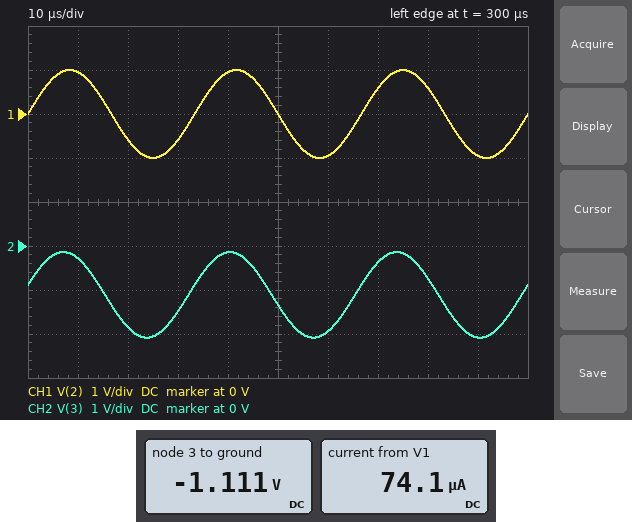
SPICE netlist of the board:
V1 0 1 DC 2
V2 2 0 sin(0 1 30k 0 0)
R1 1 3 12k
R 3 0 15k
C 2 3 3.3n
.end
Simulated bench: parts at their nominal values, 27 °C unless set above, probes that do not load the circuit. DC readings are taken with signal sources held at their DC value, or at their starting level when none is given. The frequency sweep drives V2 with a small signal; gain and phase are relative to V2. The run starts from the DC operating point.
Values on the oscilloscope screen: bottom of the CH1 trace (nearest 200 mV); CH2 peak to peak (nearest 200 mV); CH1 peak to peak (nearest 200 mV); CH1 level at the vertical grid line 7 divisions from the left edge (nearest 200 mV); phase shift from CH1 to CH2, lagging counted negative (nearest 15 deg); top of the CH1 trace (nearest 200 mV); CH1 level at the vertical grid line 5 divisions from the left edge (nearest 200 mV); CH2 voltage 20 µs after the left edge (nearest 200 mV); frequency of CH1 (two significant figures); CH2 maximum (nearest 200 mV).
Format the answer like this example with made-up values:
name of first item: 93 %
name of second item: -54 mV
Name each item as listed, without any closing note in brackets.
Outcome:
bottom of the CH1 trace: -1.0 V
CH2 peak to peak: 2.0 V
CH1 peak to peak: 2.0 V
CH1 level at the vertical grid line 7 divisions from the left edge: 600 mV
phase shift from CH1 to CH2, lagging counted negative: 15 deg
top of the CH1 trace: 1.0 V
CH1 level at the vertical grid line 5 divisions from the left edge: 0 V
CH2 voltage 20 µs after the left edge: -1.8 V
frequency of CH1: 30 kHz
CH2 maximum: -200 mV
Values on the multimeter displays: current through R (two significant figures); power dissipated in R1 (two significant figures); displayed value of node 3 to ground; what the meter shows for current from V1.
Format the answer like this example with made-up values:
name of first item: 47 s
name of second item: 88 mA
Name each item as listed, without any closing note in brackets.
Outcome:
current through R: 74 µA
power dissipated in R1: 66 µW
displayed value of node 3 to ground: -1.111 V
what the meter shows for current from V1: 74.1 µA
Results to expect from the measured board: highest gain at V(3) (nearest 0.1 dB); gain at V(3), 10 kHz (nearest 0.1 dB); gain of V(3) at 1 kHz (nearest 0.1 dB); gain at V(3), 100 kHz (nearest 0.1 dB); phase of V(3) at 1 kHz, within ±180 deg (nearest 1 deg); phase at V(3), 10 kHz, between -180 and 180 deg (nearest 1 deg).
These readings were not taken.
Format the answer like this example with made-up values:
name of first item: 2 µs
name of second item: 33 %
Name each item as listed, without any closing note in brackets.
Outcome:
highest gain at V(3): 0 dB
gain at V(3), 10 kHz: -1.8 dB
gain of V(3) at 1 kHz: -17.3 dB
gain at V(3), 100 kHz: 0 dB
phase of V(3) at 1 kHz, within ±180 deg: 82 deg
phase at V(3), 10 kHz, between -180 and 180 deg: 36 deg
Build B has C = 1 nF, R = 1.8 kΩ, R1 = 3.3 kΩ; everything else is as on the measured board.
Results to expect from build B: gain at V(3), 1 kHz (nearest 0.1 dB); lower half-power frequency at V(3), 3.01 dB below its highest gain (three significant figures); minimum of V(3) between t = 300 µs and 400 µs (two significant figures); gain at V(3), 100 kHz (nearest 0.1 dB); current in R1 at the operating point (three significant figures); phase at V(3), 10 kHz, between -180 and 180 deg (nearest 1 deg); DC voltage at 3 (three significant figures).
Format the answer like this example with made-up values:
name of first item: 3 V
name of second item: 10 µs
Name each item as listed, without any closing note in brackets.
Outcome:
gain at V(3), 1 kHz: -42.7 dB
lower half-power frequency at V(3), 3.01 dB below its highest gain: 137 kHz
minimum of V(3) between t = 300 µs and 400 µs: -920 mV
gain at V(3), 100 kHz: -4.6 dB
current in R1 at the operating point: 392 µA
phase at V(3), 10 kHz, between -180 and 180 deg: 86 deg
DC voltage at 3: -706 mV
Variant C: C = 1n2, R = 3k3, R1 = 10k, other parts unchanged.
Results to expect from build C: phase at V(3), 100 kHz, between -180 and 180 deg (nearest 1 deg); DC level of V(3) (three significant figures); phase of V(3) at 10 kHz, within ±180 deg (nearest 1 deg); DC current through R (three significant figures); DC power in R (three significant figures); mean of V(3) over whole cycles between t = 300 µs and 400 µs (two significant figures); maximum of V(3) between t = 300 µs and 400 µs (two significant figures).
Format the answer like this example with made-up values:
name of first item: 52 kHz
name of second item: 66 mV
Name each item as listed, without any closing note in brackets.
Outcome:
phase at V(3), 100 kHz, between -180 and 180 deg: 28 deg
DC level of V(3): -496 mV
phase of V(3) at 10 kHz, within ±180 deg: 79 deg
DC current through R: 150 µA
DC power in R: 74.6 µW
mean of V(3) over whole cycles between t = 300 µs and 400 µs: -500 mV
maximum of V(3) between t = 300 µs and 400 µs: -6.8 mV
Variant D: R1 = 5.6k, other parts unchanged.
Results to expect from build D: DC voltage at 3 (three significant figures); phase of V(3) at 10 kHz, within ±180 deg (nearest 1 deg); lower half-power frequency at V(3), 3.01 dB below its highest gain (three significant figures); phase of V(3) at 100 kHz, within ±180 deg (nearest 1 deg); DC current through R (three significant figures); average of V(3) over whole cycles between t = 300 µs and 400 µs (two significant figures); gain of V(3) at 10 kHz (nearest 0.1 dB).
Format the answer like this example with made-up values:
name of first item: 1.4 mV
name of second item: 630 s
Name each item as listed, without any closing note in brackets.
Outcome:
DC voltage at 3: -1.46 V
phase of V(3) at 10 kHz, within ±180 deg: 50 deg
lower half-power frequency at V(3), 3.01 dB below its highest gain: 11.8 kHz
phase of V(3) at 100 kHz, within ±180 deg: 7 deg
DC current through R: 97.1 µA
average of V(3) over whole cycles between t = 300 µs and 400 µs: -1.5 V
gain of V(3) at 10 kHz: -3.8 dB
